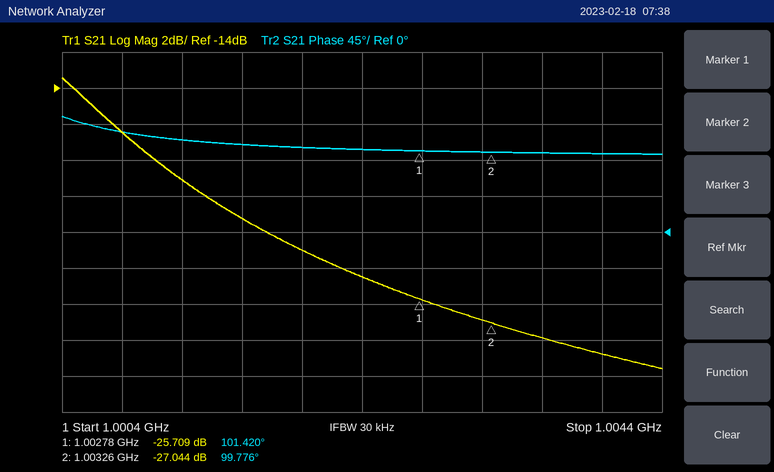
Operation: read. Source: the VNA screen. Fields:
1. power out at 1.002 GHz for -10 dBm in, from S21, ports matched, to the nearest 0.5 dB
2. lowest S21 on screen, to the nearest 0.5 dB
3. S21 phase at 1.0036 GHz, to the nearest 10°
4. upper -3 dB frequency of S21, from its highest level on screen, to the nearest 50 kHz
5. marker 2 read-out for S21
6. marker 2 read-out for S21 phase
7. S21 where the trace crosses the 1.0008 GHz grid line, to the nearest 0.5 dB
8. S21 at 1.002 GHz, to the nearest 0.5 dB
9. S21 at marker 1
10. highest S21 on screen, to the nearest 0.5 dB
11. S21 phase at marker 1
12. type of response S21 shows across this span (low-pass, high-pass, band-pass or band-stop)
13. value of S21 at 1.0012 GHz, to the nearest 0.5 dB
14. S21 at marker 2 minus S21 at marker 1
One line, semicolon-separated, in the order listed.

-33.0 dBm; -29.5 dB; 100°; 1.00080 GHz; -27.044 dB; 99.776°; -16.5 dB; -23.0 dB; -25.709 dB; -13.5 dB; 101.420°; low-pass; -19.0 dB; -1.335 dB
